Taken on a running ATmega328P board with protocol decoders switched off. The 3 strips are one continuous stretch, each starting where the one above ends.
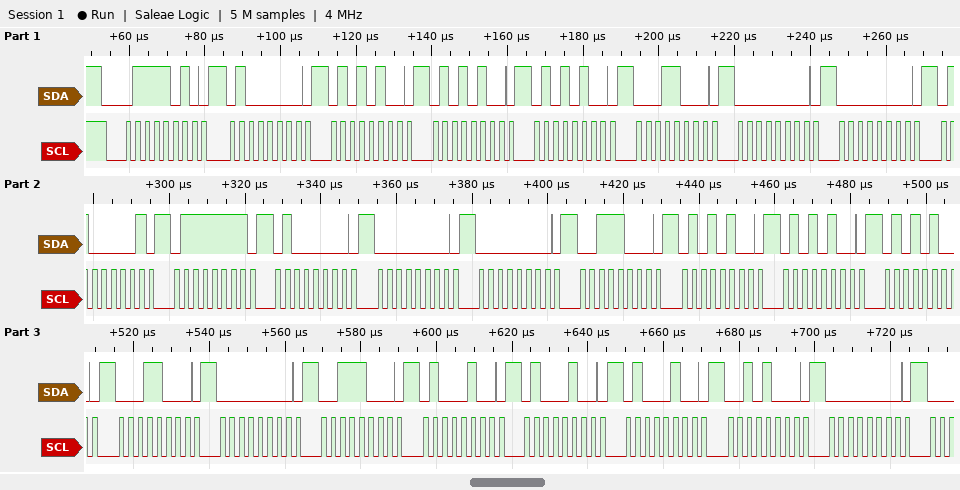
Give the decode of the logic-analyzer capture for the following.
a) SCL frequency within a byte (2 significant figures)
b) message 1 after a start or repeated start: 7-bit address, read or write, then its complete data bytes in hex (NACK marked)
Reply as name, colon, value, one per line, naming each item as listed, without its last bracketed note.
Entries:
SCL frequency within a byte: 400 kHz
message 1 after a start or repeated start: 7-bit address, read or write, then its complete data bytes in hex: 0x3D write: 40 54 54 54 18 00 00 41 7F 40 00 00 38 54 54 54 18 00 38 44 44 44 28 00
